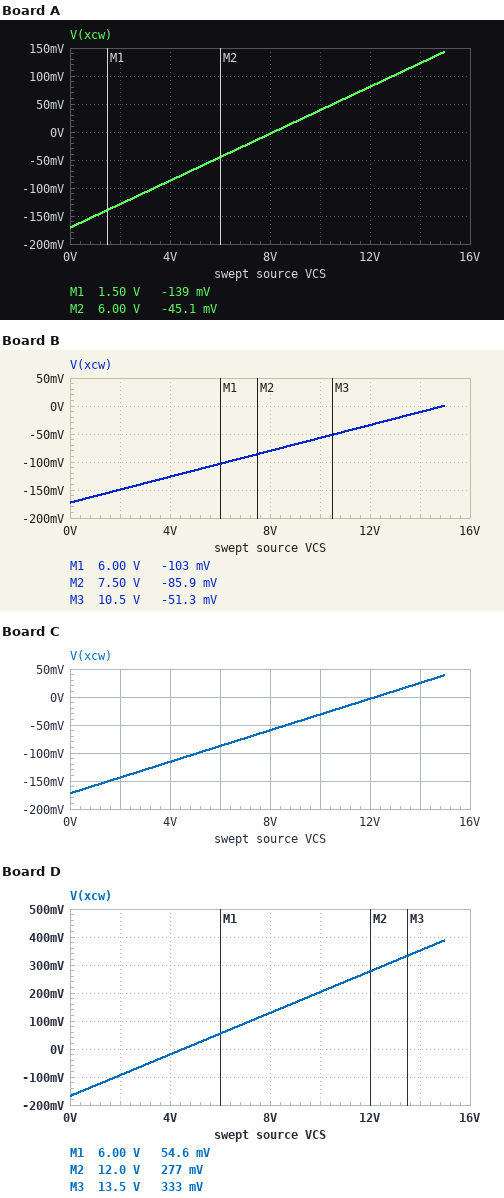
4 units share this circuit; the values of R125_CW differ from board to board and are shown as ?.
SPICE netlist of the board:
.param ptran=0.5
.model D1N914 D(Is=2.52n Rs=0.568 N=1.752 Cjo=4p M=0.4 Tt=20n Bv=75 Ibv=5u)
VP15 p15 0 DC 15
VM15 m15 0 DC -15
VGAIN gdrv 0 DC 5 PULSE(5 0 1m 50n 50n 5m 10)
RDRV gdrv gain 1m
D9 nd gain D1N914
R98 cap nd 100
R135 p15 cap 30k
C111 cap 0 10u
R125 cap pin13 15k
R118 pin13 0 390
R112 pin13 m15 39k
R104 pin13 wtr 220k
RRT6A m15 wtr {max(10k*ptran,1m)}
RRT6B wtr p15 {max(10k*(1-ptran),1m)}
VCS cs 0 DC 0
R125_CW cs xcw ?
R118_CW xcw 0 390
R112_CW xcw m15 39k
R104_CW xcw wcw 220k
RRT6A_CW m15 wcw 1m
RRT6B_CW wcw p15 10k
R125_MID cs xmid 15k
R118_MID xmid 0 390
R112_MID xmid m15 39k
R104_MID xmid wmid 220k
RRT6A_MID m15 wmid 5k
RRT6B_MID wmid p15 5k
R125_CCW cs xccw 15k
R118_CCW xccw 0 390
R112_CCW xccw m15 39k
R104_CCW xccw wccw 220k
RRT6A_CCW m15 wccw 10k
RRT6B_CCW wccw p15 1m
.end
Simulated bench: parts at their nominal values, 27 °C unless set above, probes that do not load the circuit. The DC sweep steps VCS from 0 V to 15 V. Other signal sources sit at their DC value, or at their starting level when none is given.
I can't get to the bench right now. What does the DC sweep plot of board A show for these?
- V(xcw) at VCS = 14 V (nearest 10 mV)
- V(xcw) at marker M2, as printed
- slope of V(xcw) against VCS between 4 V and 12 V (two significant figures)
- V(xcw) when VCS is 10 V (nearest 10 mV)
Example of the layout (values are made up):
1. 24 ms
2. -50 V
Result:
1. 120 mV
2. -45.1 mV
3. 0.021 V/V
4. 40 mV
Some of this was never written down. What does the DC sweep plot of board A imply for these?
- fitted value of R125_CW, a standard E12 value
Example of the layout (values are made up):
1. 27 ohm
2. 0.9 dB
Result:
1. 18 kΩ
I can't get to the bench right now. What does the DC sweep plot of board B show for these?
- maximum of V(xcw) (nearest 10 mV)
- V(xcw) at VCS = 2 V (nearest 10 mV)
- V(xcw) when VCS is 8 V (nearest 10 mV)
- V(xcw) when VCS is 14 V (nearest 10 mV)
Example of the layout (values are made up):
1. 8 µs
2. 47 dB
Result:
1. 0 V
2. -150 mV
3. -80 mV
4. -10 mV
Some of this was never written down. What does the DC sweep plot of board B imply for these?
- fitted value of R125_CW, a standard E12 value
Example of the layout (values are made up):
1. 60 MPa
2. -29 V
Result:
1. 33 kΩ
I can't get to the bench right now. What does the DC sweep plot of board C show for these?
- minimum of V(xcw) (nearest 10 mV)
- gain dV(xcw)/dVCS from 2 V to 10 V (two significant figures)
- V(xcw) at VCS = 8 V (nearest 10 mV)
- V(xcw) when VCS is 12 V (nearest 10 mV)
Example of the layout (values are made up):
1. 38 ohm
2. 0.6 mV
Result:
1. -170 mV
2. 0.014 V/V
3. -60 mV
4. 0 V
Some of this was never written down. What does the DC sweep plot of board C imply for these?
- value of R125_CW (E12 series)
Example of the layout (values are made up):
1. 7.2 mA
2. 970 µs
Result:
1. 27 kΩ
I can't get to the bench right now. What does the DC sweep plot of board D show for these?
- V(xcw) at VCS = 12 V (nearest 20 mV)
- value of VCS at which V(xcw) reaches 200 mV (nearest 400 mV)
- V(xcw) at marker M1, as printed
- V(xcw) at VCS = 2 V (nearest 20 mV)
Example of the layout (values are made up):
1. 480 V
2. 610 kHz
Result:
1. 280 mV
2. 10.0 V
3. 54.6 mV
4. -100 mV
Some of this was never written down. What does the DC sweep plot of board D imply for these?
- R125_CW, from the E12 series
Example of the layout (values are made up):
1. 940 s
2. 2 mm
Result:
1. 10 kΩ
